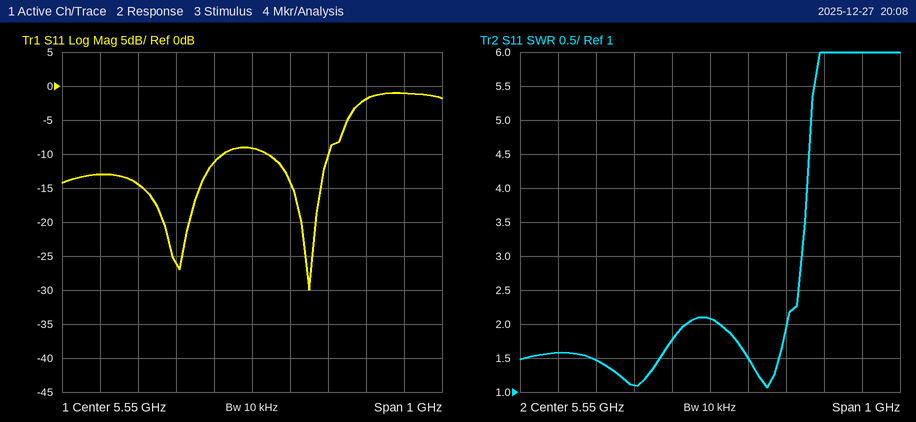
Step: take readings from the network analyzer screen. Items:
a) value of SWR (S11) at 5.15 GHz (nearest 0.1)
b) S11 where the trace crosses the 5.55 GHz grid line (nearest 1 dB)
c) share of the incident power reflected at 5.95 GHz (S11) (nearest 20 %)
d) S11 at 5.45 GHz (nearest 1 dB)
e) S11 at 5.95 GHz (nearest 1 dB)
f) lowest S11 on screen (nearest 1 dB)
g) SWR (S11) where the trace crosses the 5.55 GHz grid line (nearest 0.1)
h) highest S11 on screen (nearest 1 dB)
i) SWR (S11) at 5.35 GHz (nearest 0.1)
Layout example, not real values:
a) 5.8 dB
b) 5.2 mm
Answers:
a) 1.6
b) -9 dB
c) 80 %
d) -11 dB
e) -1 dB
f) -30 dB
g) 2.1
h) -1 dB
i) 1.1
